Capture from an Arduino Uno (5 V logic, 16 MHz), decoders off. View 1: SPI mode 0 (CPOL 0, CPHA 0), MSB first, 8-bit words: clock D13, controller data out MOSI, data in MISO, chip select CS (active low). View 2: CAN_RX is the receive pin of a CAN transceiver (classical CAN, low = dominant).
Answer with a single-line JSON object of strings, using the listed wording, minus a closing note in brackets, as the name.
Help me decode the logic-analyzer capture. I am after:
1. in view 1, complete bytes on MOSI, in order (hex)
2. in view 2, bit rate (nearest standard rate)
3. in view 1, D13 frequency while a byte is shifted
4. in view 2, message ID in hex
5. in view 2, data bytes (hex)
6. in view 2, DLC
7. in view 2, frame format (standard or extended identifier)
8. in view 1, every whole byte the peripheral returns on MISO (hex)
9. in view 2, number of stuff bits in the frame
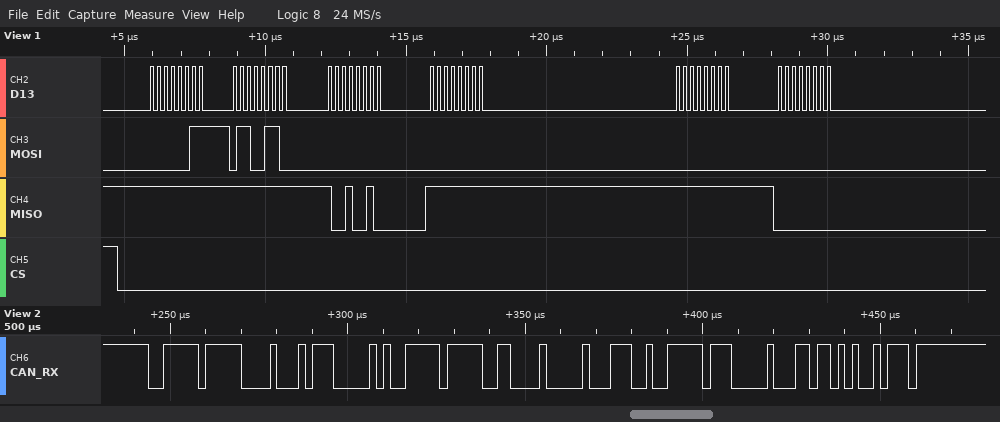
{"in view 1, complete bytes on MOSI, in order": "03 66 00 00 00 00", "in view 2, bit rate": "500 kbit/s", "in view 1, D13 frequency while a byte is shifted": "4 MHz", "in view 2, message ID in hex": "0x3FF", "in view 2, data bytes": "B8 13 FF 61 00 E4 FF 00", "in view 2, DLC": "8", "in view 2, frame format": "standard", "in view 1, every whole byte the peripheral returns on MISO": "FF FF 92 FF FF 00", "in view 2, number of stuff bits in the frame": "8"}
